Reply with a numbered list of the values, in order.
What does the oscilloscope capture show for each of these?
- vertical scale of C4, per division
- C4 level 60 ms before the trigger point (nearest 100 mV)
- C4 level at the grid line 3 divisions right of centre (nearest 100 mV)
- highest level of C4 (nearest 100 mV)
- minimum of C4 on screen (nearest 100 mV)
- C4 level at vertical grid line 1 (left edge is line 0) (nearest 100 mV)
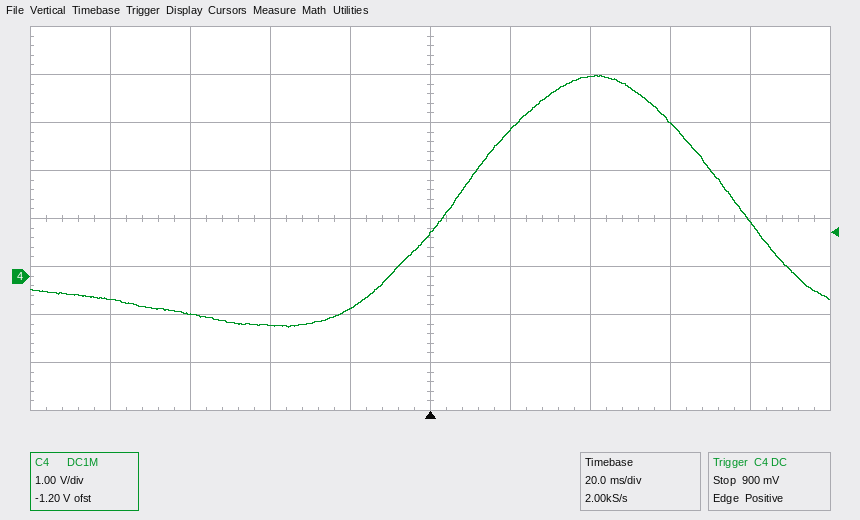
1. 1 V
2. -800 mV
3. 3.2 V
4. 4.2 V
5. -1.1 V
6. -500 mV
